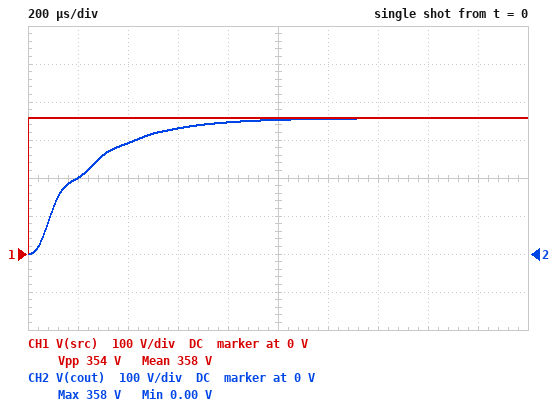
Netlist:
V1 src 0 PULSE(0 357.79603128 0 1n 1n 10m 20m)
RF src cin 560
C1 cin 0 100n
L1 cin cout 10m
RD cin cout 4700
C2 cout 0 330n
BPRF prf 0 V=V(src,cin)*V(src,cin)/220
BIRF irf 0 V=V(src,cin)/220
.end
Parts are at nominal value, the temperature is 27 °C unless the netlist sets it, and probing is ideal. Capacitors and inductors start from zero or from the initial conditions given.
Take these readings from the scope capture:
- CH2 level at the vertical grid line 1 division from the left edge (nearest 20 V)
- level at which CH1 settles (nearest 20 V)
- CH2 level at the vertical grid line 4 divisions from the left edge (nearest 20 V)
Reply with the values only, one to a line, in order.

200 V
360 V
340 V
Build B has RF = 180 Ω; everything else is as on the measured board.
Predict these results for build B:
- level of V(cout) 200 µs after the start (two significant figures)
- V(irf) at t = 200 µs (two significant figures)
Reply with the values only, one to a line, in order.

390 V
150 mV
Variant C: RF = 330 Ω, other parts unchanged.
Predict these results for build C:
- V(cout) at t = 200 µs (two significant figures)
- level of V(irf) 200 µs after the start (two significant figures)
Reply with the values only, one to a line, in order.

280 V
390 mV
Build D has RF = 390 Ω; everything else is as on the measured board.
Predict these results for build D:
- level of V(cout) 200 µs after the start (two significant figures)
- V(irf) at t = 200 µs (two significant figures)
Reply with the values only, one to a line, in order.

260 V
470 mV
